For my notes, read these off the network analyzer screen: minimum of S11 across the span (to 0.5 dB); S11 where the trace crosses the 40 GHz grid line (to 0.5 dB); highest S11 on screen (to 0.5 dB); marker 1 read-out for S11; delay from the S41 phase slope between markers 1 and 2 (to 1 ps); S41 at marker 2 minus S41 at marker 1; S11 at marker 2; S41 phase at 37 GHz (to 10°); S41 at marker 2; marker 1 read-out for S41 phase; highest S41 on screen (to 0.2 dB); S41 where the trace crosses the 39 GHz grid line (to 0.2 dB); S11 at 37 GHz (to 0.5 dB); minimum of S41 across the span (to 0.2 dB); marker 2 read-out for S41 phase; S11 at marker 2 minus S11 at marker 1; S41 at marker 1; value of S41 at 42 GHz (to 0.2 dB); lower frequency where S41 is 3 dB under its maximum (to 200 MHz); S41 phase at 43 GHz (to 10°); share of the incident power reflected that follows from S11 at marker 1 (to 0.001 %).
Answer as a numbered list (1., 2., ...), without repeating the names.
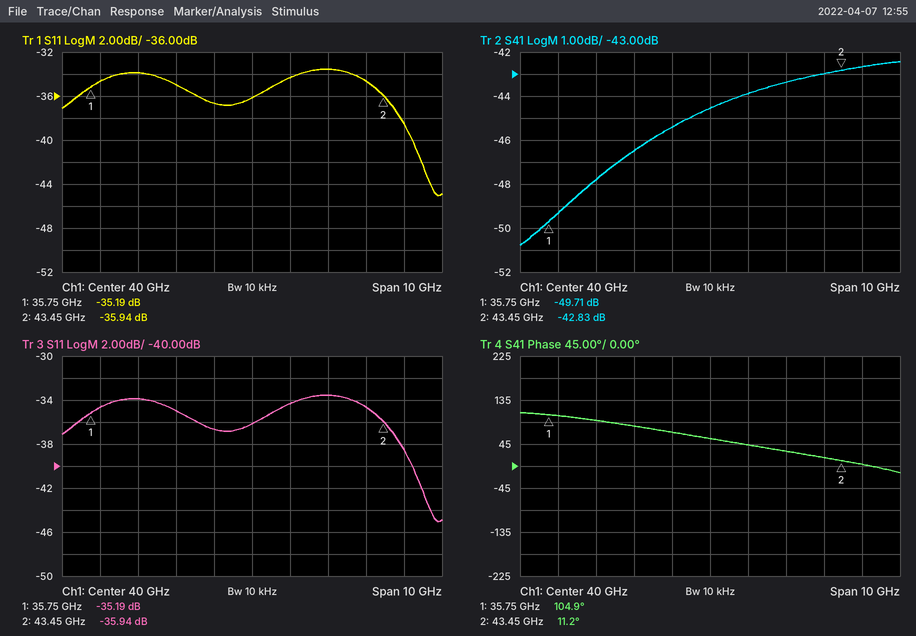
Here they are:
1. -45.0 dB
2. -36.0 dB
3. -33.5 dB
4. -35.19 dB
5. 34 ps
6. 6.88 dB
7. -35.94 dB
8. 90°
9. -42.83 dB
10. 104.9°
11. -42.4 dB
12. -45.4 dB
13. -34.0 dB
14. -50.8 dB
15. 11.2°
16. -0.75 dB
17. -49.71 dB
18. -43.4 dB
19. 39.0 GHz
20. 20°
21. 0.030 %
